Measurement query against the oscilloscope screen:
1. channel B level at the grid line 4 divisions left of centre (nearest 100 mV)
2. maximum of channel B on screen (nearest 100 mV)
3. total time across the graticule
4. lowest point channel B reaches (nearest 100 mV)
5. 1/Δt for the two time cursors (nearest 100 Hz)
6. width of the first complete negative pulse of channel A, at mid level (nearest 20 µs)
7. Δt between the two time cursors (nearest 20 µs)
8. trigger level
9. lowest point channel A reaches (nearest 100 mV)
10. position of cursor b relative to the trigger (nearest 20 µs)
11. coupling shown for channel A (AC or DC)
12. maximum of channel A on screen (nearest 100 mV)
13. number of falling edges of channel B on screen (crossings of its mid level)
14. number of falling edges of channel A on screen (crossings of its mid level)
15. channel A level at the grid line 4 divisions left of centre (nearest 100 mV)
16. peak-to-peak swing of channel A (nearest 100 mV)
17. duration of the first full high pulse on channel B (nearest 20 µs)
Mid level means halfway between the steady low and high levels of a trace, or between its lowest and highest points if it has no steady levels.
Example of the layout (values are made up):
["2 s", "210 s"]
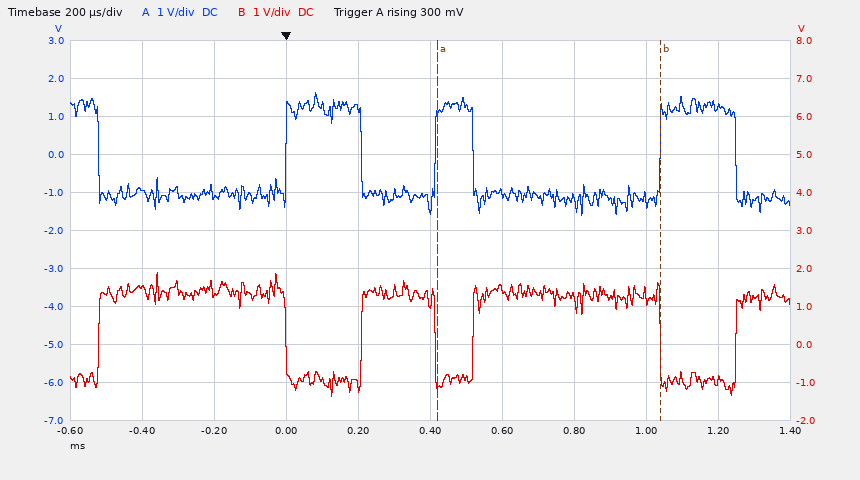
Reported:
["1.5 V", "1.9 V", "2 ms", "-1.4 V", "1.6 kHz", "520 µs", "620 µs", "300 mV", "-1.6 V", "+1.04 ms", "DC", "1.6 V", "3", "4", "-900 mV", "3.2 V", "520 µs"]
